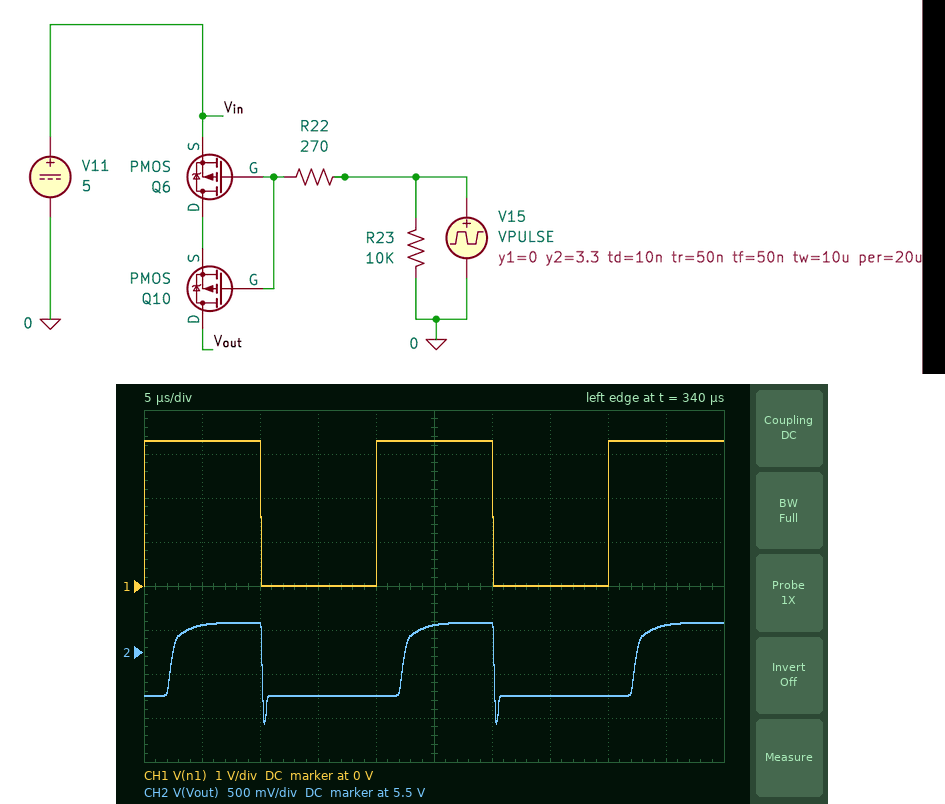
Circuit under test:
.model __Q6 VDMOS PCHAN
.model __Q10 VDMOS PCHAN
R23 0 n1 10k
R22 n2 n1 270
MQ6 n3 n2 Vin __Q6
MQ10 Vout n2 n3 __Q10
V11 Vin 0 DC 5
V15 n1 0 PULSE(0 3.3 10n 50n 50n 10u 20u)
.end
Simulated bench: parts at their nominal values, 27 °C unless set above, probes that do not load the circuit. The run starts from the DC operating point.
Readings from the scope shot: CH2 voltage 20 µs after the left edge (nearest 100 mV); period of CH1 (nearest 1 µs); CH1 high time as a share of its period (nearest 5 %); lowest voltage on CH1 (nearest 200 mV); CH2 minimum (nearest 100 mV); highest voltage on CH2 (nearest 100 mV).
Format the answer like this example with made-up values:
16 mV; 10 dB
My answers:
5.0 V; 20 µs; 50 %; 0 V; 4.7 V; 5.8 V
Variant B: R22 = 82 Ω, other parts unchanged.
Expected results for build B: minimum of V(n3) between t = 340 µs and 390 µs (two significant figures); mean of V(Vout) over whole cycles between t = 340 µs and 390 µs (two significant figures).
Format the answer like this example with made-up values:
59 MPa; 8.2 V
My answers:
4.5 V; 5.4 V
